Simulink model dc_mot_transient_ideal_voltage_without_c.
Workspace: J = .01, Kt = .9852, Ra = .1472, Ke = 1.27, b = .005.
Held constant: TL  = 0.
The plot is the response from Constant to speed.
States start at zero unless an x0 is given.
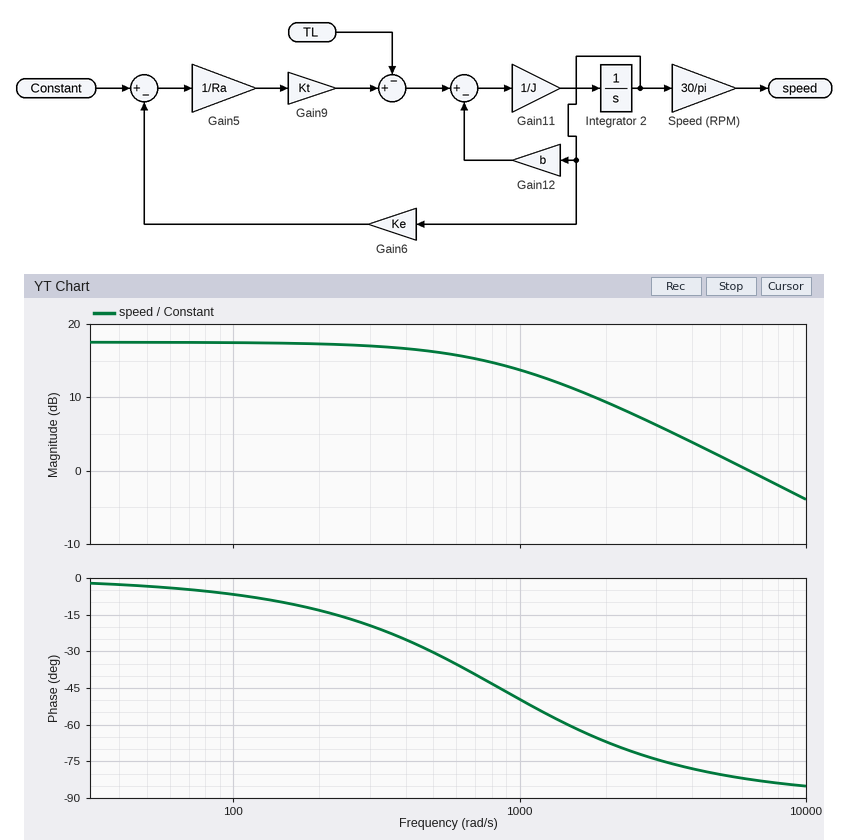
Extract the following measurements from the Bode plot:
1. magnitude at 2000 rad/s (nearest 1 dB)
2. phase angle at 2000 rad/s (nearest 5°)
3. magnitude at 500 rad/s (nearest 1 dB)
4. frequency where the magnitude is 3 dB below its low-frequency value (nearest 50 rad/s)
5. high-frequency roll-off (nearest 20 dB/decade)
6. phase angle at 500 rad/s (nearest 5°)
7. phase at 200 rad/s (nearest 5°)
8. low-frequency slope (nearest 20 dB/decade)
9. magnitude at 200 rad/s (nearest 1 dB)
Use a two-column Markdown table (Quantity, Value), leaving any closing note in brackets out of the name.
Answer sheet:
| Quantity | Value |
|---|---|
| magnitude at 2000 rad/s | 9 dB |
| phase angle at 2000 rad/s | -65° |
| magnitude at 500 rad/s | 16 dB |
| frequency where the magnitude is 3 dB below its low-frequency value | 850 rad/s |
| high-frequency roll-off | -20 dB/decade |
| phase angle at 500 rad/s | -30° |
| phase at 200 rad/s | -15° |
| low-frequency slope | 0 dB/decade |
| magnitude at 200 rad/s | 17 dB |
